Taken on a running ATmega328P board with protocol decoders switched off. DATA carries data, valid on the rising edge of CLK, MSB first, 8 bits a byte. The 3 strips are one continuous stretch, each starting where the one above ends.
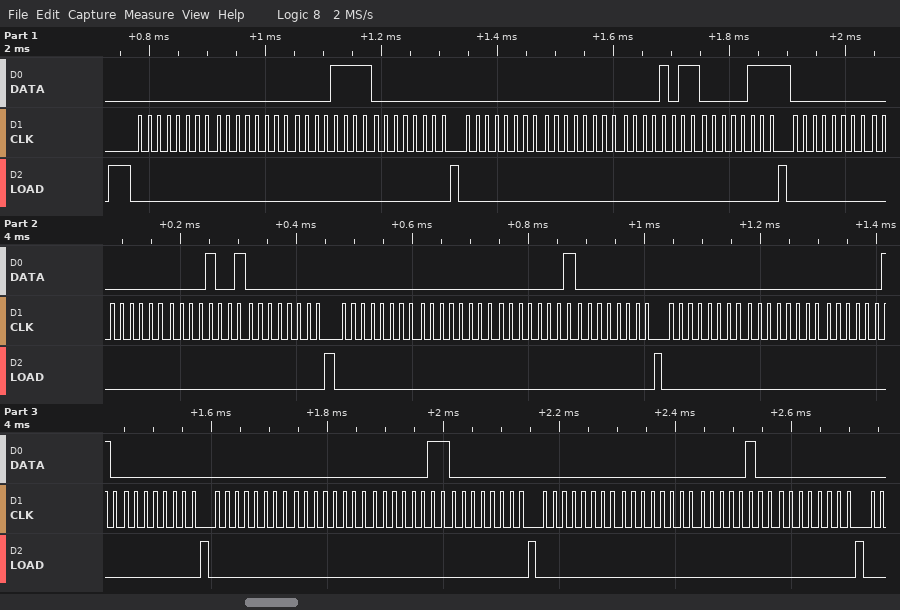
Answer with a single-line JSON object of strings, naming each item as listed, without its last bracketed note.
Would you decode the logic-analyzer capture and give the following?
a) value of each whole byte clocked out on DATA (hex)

{"value of each whole byte clocked out on DATA": "0x00 0x00 0x0F 0x00 0x00 0x00 0x0B 0x07 0x00 0x00 0x09 0x00 0x00 0x00 0x01 0x00 0x00 0x00 0x02 0x00 0x00 0x00 0x03 0x00 0x00 0x00 0x04 0x00"}
